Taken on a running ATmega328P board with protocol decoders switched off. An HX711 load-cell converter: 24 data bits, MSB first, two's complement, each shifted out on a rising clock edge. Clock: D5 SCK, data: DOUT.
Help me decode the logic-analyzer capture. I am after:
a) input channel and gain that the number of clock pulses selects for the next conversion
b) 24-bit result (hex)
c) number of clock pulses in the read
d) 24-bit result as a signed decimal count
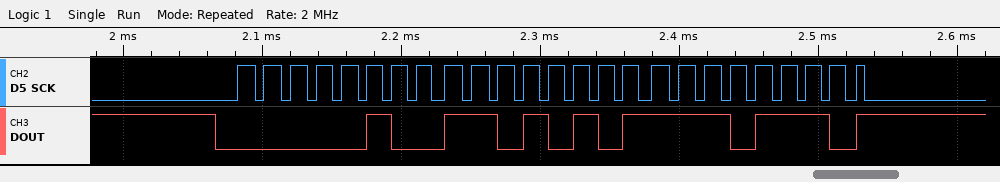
channel A, gain 128
0x04D5EE
25
316910
